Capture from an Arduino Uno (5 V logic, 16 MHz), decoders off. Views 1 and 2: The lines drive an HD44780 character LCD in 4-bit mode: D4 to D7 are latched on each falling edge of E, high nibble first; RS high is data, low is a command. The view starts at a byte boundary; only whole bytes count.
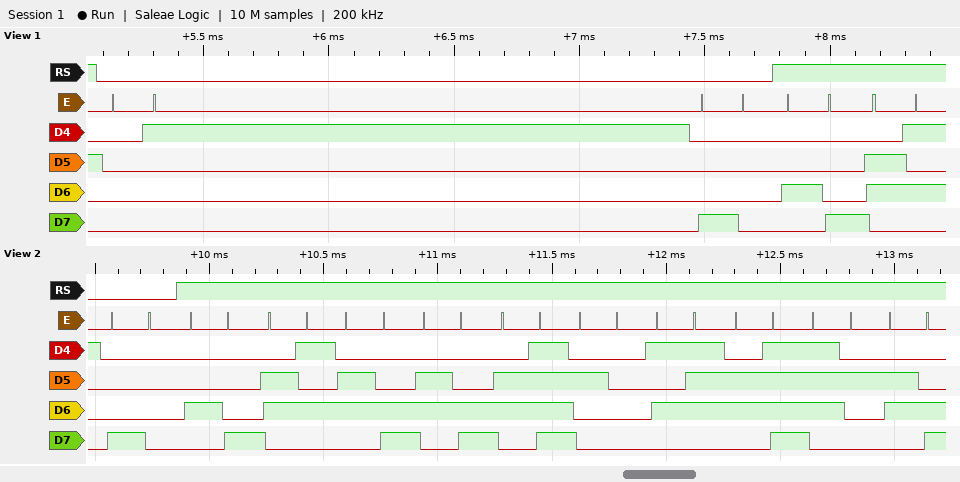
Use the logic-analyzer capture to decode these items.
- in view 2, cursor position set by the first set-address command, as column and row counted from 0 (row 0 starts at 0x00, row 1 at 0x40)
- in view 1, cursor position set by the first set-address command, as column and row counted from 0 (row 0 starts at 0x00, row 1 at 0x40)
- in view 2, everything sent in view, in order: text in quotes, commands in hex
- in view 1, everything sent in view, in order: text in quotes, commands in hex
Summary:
column 0, row 0
column 0, row 0
0x80 "Hello Worl"
0x01 0x80 "He"
